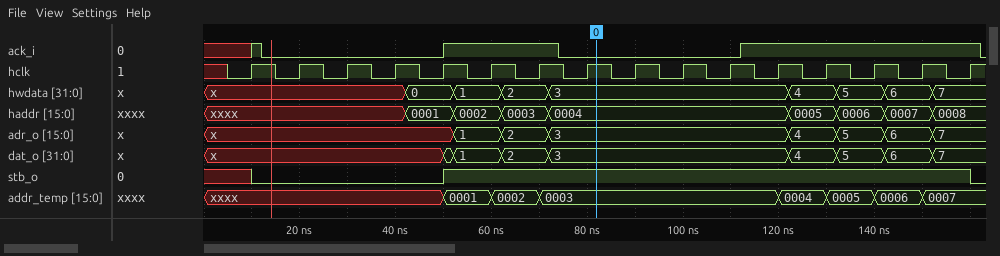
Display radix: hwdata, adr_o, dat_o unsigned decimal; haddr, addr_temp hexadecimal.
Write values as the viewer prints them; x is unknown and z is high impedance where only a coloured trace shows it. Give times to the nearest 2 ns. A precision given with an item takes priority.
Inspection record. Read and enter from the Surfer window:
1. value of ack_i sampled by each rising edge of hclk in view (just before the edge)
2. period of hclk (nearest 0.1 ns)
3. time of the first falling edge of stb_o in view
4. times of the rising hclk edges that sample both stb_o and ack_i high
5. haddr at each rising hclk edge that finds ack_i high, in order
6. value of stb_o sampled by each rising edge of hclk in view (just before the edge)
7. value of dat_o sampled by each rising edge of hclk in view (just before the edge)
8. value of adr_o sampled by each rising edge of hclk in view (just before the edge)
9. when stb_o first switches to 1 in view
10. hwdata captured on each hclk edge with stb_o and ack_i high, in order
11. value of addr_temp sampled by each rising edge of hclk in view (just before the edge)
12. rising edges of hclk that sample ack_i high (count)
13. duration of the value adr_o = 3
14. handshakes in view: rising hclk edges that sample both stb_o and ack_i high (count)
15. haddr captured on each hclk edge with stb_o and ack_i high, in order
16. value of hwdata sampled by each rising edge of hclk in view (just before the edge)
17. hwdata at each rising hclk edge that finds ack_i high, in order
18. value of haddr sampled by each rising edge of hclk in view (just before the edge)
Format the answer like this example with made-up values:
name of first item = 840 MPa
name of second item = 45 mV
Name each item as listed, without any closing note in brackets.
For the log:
value of ack_i sampled by each rising edge of hclk in view = x 0 0 0 0 1 1 0 0 0 0 1 1 1 1 1
period of hclk = 10 ns
time of the first falling edge of stb_o in view = 160 ns
times of the rising hclk edges that sample both stb_o and ack_i high = 60 ns, 70 ns, 120 ns, 130 ns, 140 ns, 150 ns, 160 ns
haddr at each rising hclk edge that finds ack_i high, in order = 0002, 0003, 0004, 0005, 0006, 0007, 0008
value of stb_o sampled by each rising edge of hclk in view = x 0 0 0 0 1 1 1 1 1 1 1 1 1 1 1
value of dat_o sampled by each rising edge of hclk in view = x, x, x, x, x, 1, 2, 3, 3, 3, 3, 3, 4, 5, 6, 7
value of adr_o sampled by each rising edge of hclk in view = x, x, x, x, x, 1, 2, 3, 3, 3, 3, 3, 4, 5, 6, 7
when stb_o first switches to 1 in view = 50 ns
hwdata captured on each hclk edge with stb_o and ack_i high, in order = 1, 2, 3, 4, 5, 6, 7
value of addr_temp sampled by each rising edge of hclk in view = xxxx, xxxx, xxxx, xxxx, xxxx, 0001, 0002, 0003, 0003, 0003, 0003, 0003, 0004, 0005, 0006, 0007
rising edges of hclk that sample ack_i high = 7
duration of the value adr_o = 3 = 50 ns
handshakes in view: rising hclk edges that sample both stb_o and ack_i high = 7
haddr captured on each hclk edge with stb_o and ack_i high, in order = 0002, 0003, 0004, 0005, 0006, 0007, 0008
value of hwdata sampled by each rising edge of hclk in view = x, x, x, x, 0, 1, 2, 3, 3, 3, 3, 3, 4, 5, 6, 7
hwdata at each rising hclk edge that finds ack_i high, in order = 1, 2, 3, 4, 5, 6, 7
value of haddr sampled by each rising edge of hclk in view = xxxx, xxxx, xxxx, xxxx, 0001, 0002, 0003, 0004, 0004, 0004, 0004, 0004, 0005, 0006, 0007, 0008
